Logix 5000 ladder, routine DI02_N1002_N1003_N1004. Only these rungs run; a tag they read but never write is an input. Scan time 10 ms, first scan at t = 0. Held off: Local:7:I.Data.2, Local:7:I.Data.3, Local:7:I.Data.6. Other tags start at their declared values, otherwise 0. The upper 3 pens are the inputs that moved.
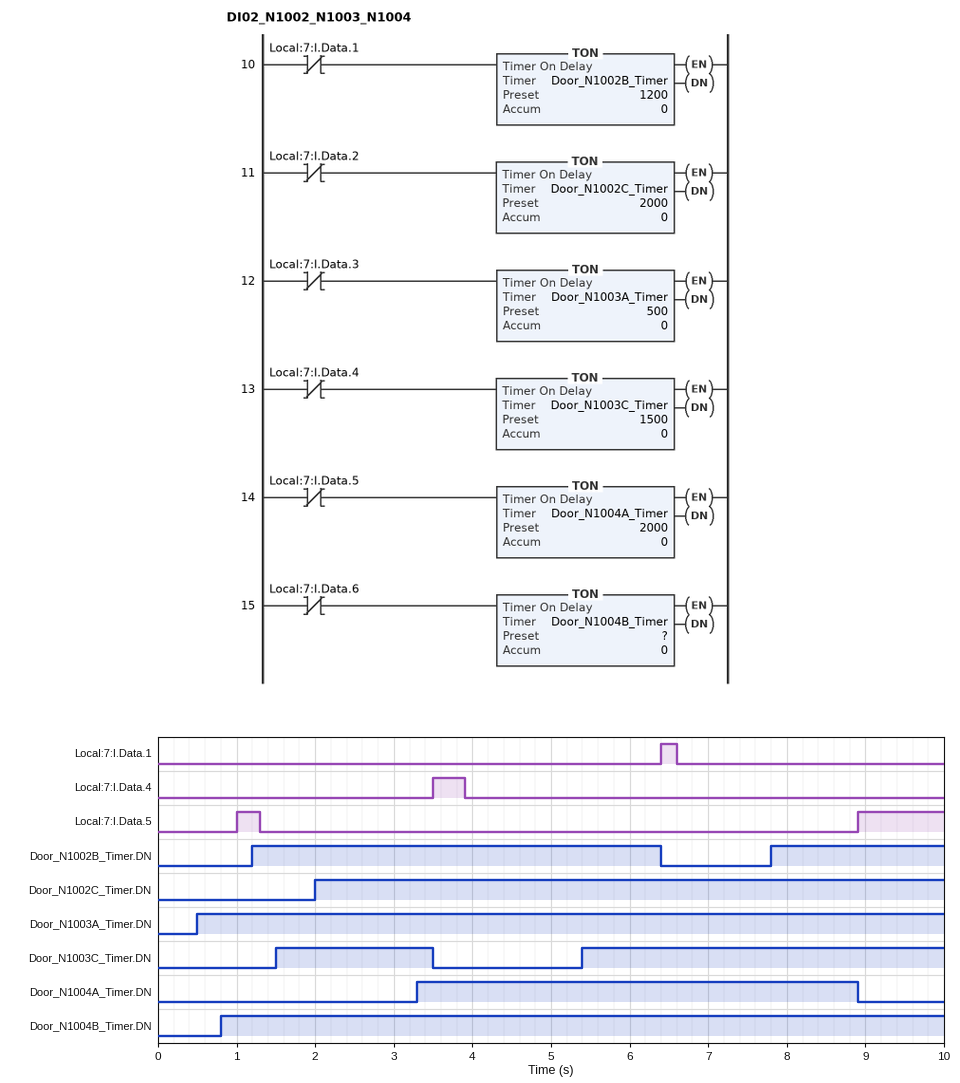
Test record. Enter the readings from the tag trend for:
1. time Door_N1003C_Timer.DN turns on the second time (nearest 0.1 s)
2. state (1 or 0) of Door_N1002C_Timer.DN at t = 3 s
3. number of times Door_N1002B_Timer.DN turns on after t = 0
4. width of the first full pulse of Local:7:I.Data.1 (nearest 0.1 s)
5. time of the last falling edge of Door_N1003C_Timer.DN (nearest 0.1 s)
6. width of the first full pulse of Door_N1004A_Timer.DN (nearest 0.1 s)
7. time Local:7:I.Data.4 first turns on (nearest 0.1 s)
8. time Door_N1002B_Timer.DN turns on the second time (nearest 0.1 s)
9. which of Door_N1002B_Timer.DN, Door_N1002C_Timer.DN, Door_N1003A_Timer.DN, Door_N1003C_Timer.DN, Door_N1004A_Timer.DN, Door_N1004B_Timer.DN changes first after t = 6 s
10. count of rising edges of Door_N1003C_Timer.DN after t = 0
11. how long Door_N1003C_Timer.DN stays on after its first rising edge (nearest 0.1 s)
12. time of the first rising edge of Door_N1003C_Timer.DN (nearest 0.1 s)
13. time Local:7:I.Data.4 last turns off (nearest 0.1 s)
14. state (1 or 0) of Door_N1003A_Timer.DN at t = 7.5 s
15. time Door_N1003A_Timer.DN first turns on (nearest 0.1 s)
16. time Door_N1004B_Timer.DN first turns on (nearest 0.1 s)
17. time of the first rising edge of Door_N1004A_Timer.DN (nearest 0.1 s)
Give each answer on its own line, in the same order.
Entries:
5.4 s
1
2
0.2 s
3.5 s
5.6 s
3.5 s
7.8 s
Door_N1002B_Timer.DN
2
2.0 s
1.5 s
3.9 s
1
0.5 s
0.8 s
3.3 s
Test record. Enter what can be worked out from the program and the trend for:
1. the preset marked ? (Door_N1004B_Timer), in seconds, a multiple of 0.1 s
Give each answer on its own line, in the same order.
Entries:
0.8 s
